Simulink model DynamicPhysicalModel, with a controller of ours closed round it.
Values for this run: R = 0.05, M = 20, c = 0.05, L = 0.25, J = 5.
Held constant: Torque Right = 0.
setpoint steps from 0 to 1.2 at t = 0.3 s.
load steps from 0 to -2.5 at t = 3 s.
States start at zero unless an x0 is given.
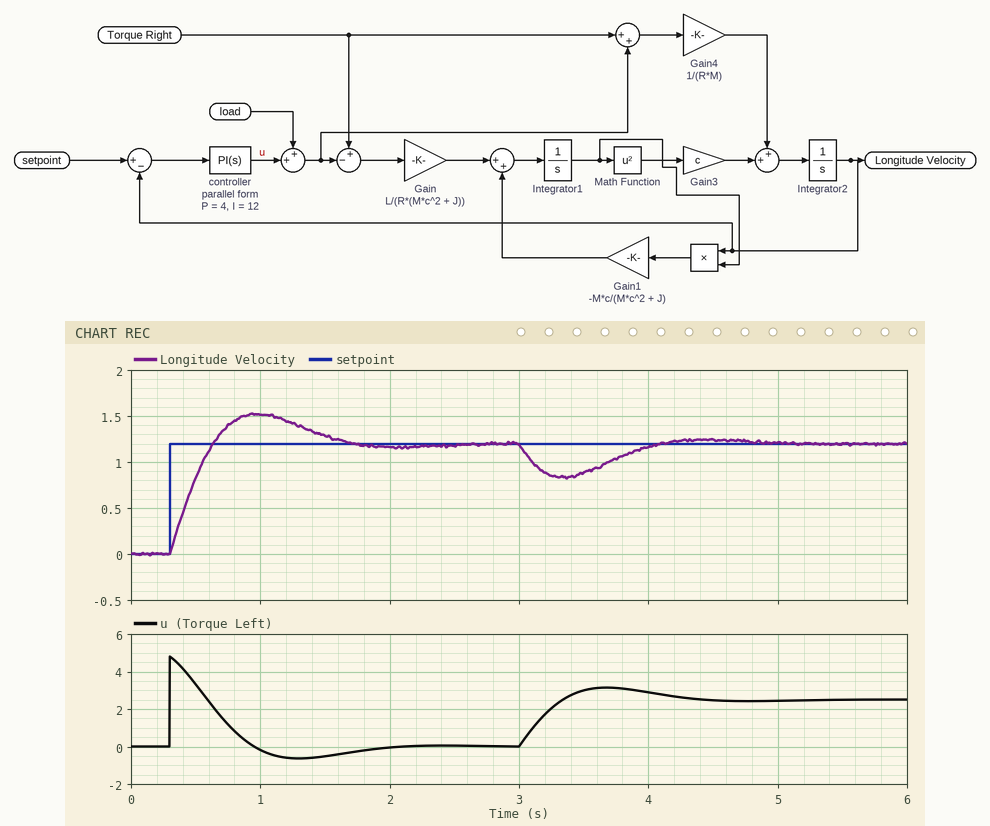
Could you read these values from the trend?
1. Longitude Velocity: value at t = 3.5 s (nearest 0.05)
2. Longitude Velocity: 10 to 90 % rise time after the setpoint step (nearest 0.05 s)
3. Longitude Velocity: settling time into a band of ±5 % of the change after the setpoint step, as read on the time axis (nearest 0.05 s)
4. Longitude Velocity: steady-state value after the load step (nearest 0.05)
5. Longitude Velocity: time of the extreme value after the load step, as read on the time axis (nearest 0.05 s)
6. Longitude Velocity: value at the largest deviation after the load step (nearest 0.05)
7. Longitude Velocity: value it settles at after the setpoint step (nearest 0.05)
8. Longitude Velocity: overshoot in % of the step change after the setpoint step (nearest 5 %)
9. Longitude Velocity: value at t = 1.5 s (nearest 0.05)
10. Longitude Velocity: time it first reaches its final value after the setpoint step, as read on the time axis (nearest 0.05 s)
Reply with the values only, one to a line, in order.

0.90
0.25 s
1.55 s
1.20
3.35 s
0.85
1.20
25 %
1.30
0.65 s
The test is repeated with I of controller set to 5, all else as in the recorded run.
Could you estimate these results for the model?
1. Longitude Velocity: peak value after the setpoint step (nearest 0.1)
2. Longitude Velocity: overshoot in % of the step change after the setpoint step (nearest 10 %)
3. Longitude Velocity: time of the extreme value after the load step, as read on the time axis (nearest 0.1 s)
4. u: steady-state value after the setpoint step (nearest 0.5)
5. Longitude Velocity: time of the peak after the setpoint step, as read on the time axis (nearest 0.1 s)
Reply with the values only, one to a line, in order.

1.4
20 %
3.5 s
0.0
1.2 s
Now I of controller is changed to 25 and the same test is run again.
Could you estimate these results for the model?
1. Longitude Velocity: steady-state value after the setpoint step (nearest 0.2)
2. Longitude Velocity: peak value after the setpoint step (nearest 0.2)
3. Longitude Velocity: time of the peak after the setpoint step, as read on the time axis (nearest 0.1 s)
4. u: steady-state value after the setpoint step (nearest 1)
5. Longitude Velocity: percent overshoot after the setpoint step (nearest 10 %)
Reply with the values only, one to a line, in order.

1.2
1.6
0.8 s
0
40 %
